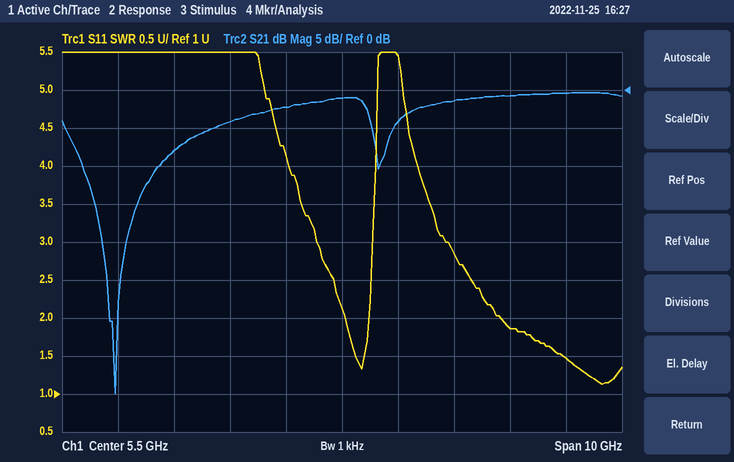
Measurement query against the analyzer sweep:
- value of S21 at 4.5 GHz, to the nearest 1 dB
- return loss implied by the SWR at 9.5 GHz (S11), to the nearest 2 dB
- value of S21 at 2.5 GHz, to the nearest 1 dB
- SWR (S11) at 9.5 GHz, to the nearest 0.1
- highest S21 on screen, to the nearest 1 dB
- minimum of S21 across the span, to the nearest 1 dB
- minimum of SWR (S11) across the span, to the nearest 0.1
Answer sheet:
-2 dB
14 dB
-8 dB
1.5
0 dB
-40 dB
1.1
